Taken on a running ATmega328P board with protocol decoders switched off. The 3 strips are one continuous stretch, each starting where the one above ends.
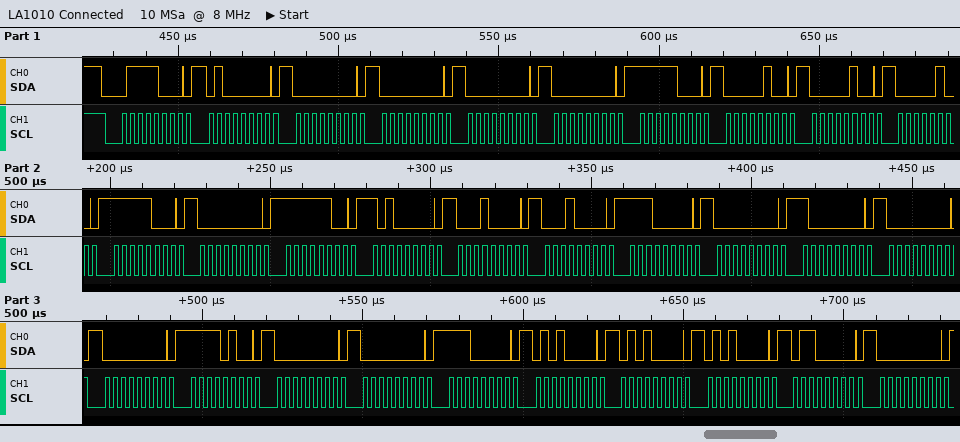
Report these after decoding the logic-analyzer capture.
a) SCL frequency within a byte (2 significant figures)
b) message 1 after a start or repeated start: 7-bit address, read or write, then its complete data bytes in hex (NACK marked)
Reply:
400 kHz
0x3C write: 40 00 00 00 00 F8 04 04 04 F8 00 FC A0 10 10 E0 00 80 00 00 F4 00 00 E0 50 50 50 60 00
